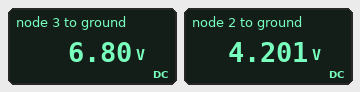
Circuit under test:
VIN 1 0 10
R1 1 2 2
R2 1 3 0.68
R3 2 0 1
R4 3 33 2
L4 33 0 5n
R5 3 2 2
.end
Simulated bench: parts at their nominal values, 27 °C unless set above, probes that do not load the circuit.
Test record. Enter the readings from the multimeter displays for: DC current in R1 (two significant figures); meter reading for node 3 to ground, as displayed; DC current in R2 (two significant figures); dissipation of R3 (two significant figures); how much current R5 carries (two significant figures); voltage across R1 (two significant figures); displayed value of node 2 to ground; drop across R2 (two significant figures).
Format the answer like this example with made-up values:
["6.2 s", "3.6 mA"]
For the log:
["2.9 A", "6.80 V", "4.7 A", "18 W", "1.3 A", "5.8 V", "4.201 V", "3.2 V"]
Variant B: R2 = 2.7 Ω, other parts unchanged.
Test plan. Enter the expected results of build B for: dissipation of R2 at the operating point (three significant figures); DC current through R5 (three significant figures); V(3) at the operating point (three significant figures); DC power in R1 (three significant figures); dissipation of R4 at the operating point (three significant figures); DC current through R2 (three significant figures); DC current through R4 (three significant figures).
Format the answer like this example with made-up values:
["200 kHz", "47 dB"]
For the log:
["13.4 W", "242 mA", "3.98 V", "21.2 W", "7.91 W", "2.23 A", "1.99 A"]
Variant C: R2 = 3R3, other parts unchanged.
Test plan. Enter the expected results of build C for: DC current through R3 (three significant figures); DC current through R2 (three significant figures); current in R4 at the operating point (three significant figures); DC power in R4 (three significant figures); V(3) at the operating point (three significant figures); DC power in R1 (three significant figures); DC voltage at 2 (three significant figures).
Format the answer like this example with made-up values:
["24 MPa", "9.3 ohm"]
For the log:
["3.41 A", "1.93 A", "1.82 A", "6.60 W", "3.63 V", "21.7 W", "3.41 V"]
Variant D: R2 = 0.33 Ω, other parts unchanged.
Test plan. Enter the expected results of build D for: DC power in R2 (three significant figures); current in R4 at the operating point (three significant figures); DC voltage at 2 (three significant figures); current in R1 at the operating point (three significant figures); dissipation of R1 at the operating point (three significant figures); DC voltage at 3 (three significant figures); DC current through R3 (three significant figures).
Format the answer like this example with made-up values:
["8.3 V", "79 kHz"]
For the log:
["11.2 W", "4.04 A", "4.52 V", "2.74 A", "15.0 W", "8.08 V", "4.52 A"]
